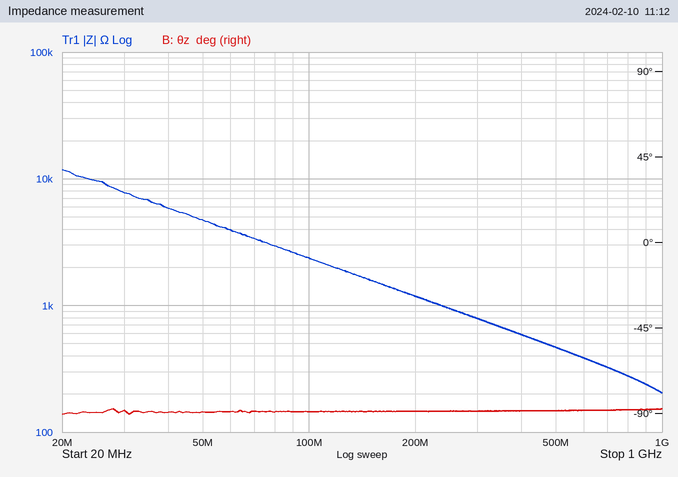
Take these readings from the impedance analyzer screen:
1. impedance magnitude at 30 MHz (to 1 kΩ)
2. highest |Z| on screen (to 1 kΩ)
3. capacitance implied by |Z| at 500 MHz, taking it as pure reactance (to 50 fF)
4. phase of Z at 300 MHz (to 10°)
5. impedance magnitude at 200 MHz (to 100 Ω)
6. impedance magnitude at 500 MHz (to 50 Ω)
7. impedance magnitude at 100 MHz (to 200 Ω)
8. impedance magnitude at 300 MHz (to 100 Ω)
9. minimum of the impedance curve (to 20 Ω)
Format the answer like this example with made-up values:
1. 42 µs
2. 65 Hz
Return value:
1. 8 kΩ
2. 12 kΩ
3. 700 fF
4. -90°
5. 1.2 kΩ
6. 450 Ω
7. 2.4 kΩ
8. 800 Ω
9. 200 Ω
